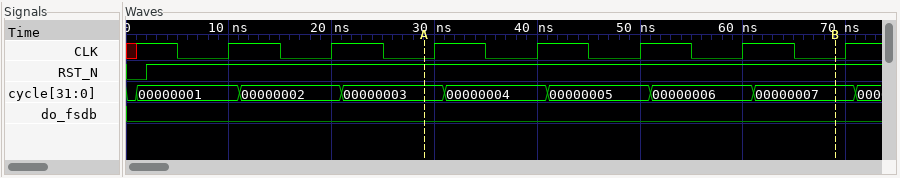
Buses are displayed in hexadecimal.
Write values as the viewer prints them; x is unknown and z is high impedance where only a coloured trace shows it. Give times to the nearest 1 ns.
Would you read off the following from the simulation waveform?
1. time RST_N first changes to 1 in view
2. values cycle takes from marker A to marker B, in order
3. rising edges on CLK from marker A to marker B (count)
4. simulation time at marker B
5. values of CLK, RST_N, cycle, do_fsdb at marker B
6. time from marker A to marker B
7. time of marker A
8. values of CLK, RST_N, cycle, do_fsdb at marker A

2 ns
00000003, 00000004, 00000005, 00000006, 00000007
4
69 ns
CLK=0, RST_N=1, cycle=00000007, do_fsdb=0
40 ns
29 ns
CLK=0, RST_N=1, cycle=00000003, do_fsdb=0
